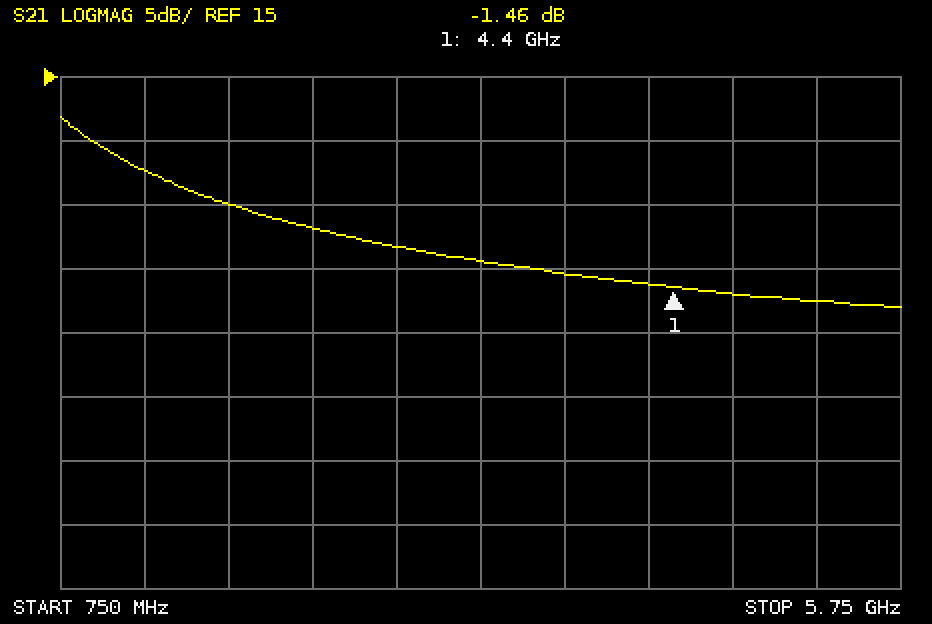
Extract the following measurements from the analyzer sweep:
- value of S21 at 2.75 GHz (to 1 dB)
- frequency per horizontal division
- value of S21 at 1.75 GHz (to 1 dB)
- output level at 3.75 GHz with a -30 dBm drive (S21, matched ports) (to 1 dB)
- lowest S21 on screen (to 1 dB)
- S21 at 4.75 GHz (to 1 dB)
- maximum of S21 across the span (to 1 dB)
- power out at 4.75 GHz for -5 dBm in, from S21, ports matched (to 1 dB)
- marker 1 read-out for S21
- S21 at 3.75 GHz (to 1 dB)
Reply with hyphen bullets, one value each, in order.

- 2 dB
- 500 MHz
- 5 dB
- -30 dBm
- -3 dB
- -2 dB
- 12 dB
- -7 dBm
- -1.46 dB
- 0 dB
